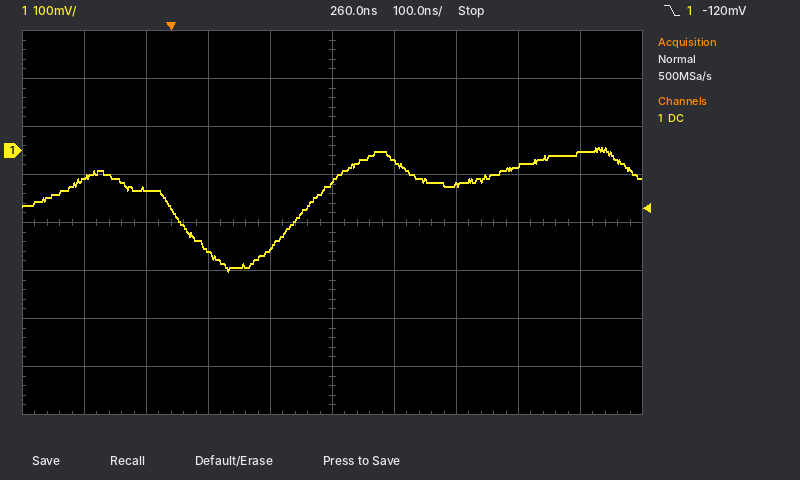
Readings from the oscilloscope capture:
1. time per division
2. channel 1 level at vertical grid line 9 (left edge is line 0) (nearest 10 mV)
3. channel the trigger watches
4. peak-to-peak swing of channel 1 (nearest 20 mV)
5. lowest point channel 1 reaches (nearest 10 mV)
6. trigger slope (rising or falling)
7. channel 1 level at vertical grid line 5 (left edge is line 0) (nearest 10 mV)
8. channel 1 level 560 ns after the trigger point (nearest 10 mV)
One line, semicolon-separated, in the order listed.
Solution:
100 ns; 0 mV; channel 1; 260 mV; -250 mV; falling; -70 mV; -30 mV
